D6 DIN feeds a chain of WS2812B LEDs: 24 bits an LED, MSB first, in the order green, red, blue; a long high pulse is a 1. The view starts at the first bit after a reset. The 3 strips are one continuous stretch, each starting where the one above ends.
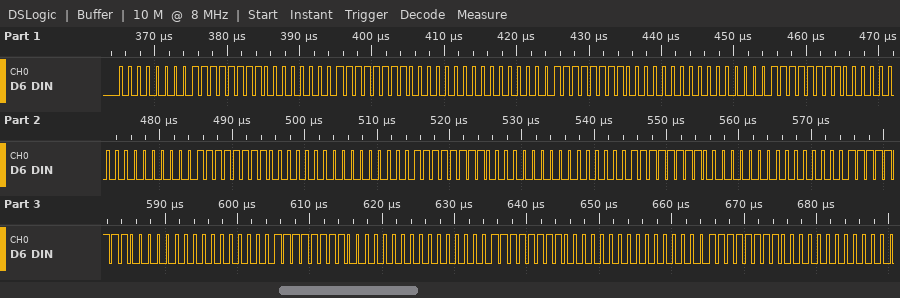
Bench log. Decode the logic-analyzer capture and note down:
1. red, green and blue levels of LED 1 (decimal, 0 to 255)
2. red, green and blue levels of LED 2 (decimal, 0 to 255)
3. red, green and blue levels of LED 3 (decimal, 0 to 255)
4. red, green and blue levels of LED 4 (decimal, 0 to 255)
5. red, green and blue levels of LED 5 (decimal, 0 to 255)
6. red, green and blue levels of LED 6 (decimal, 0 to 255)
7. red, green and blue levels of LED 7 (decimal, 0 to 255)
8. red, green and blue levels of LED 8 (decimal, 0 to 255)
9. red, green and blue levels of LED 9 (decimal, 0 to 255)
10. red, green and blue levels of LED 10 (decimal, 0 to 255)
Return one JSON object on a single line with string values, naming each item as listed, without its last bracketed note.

{"red, green and blue levels of LED 1": "255, 0, 0", "red, green and blue levels of LED 2": "0, 255, 0", "red, green and blue levels of LED 3": "0, 255, 0", "red, green and blue levels of LED 4": "0, 255, 0", "red, green and blue levels of LED 5": "0, 255, 0", "red, green and blue levels of LED 6": "0, 255, 0", "red, green and blue levels of LED 7": "0, 255, 0", "red, green and blue levels of LED 8": "0, 255, 0", "red, green and blue levels of LED 9": "0, 255, 0", "red, green and blue levels of LED 10": "0, 255, 0"}
